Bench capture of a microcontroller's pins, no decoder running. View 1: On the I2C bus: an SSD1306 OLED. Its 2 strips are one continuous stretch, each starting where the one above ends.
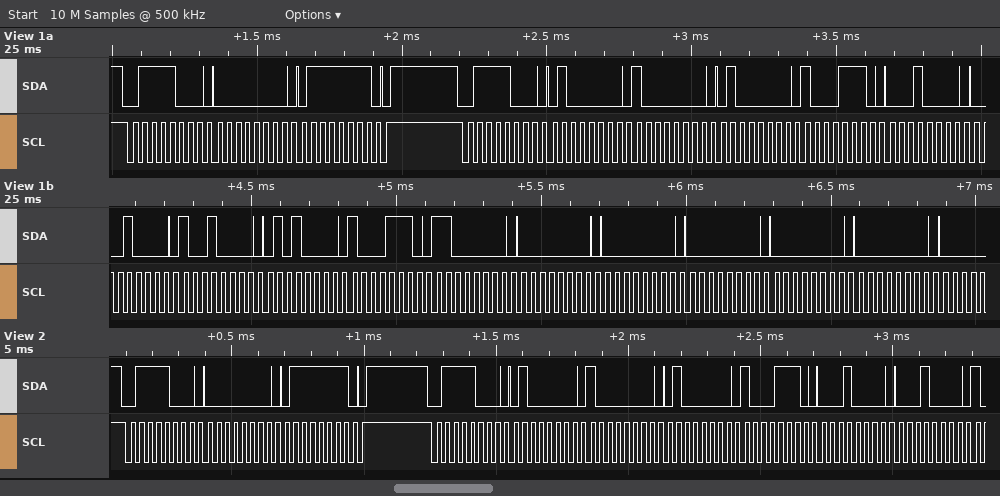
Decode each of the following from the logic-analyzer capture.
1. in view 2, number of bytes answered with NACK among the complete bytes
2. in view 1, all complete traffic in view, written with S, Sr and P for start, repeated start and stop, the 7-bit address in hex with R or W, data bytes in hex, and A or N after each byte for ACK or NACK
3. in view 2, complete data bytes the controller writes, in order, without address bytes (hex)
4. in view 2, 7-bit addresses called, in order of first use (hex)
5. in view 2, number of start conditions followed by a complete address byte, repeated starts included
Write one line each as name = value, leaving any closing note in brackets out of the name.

in view 2, number of bytes answered with NACK among the complete bytes = 0
in view 1, all complete traffic in view, written with S, Sr and P for start, repeated start and stop, the 7-bit address in hex with R or W, data bytes in hex, and A or N after each byte for ACK or NACK = S 3CW A 00 A 7F A P S 3CW A 40 A 80 A 40 A 8E A 10 A 10 A 90 A 50 A 8E A C0 A 00 A 00 A 00 A 00 A 00 A
in view 2, complete data bytes the controller writes, in order, without address bytes = 00 7F 40 80 40 8E 10 10
in view 2, 7-bit addresses called, in order of first use = 0x3C
in view 2, number of start conditions followed by a complete address byte, repeated starts included = 2
